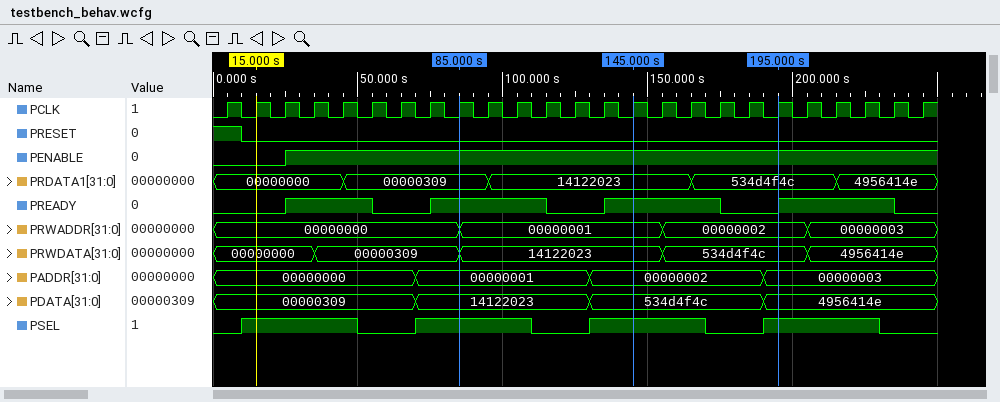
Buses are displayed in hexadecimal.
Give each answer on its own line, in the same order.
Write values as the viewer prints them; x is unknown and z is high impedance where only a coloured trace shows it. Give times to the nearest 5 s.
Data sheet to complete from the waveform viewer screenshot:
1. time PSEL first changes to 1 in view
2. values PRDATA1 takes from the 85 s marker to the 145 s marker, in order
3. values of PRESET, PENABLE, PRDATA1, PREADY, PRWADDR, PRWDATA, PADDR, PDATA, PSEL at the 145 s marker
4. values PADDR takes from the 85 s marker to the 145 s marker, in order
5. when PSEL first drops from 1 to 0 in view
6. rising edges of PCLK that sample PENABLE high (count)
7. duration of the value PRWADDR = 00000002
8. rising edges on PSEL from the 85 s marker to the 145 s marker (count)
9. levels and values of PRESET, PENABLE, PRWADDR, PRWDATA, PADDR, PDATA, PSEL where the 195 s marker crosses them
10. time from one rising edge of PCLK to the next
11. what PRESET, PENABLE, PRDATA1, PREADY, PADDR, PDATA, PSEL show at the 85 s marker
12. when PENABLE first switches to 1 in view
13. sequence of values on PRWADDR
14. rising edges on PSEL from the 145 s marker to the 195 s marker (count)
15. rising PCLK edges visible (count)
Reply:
10 s
00000309, 14122023
PRESET=0, PENABLE=1, PRDATA1=14122023, PREADY=1, PRWADDR=00000001, PRWDATA=14122023, PADDR=00000002, PDATA=534d4f4c, PSEL=1
00000001, 00000002
50 s
22
50 s
1
PRESET=0, PENABLE=1, PRWADDR=00000002, PRWDATA=534d4f4c, PADDR=00000003, PDATA=4956414e, PSEL=1
10 s
PRESET=0, PENABLE=1, PRDATA1=00000309, PREADY=1, PADDR=00000001, PDATA=14122023, PSEL=1
25 s
00000000, 00000001, 00000002, 00000003
1
25
